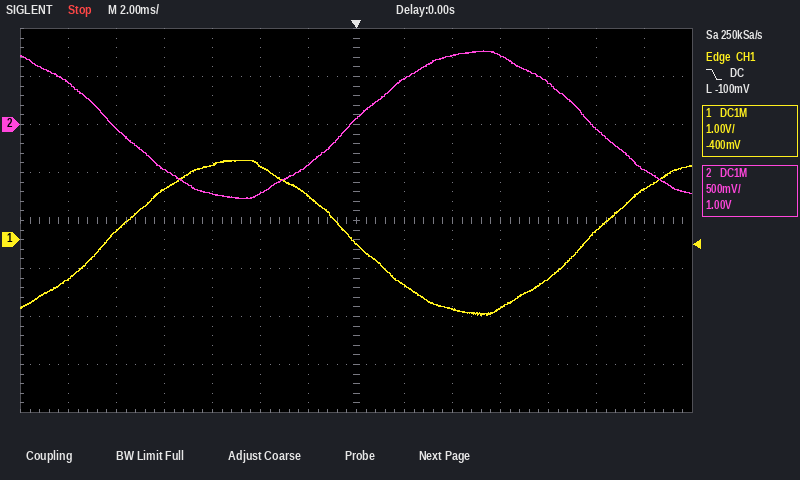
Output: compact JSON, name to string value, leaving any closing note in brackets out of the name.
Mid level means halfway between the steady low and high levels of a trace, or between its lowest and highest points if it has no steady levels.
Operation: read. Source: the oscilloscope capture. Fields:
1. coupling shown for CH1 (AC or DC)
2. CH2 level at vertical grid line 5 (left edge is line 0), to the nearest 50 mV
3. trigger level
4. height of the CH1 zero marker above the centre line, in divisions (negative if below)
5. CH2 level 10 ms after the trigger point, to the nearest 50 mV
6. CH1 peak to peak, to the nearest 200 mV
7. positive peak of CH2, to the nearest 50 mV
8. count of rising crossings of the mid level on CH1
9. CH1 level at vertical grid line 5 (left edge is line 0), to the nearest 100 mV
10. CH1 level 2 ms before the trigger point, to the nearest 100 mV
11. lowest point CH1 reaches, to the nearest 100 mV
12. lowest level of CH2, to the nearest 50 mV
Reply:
{"coupling shown for CH1": "DC", "CH2 level at vertical grid line 5 (left edge is line 0), to the nearest 50 mV": "-700 mV", "trigger level": "-100 mV", "height of the CH1 zero marker above the centre line, in divisions": "-0.4 div", "CH2 level 10 ms after the trigger point, to the nearest 50 mV": "-50 mV", "CH1 peak to peak, to the nearest 200 mV": "3.2 V", "positive peak of CH2, to the nearest 50 mV": "750 mV", "count of rising crossings of the mid level on CH1": "2", "CH1 level at vertical grid line 5 (left edge is line 0), to the nearest 100 mV": "1.5 V", "CH1 level 2 ms before the trigger point, to the nearest 100 mV": "900 mV", "lowest point CH1 reaches, to the nearest 100 mV": "-1.6 V", "lowest level of CH2, to the nearest 50 mV": "-750 mV"}
